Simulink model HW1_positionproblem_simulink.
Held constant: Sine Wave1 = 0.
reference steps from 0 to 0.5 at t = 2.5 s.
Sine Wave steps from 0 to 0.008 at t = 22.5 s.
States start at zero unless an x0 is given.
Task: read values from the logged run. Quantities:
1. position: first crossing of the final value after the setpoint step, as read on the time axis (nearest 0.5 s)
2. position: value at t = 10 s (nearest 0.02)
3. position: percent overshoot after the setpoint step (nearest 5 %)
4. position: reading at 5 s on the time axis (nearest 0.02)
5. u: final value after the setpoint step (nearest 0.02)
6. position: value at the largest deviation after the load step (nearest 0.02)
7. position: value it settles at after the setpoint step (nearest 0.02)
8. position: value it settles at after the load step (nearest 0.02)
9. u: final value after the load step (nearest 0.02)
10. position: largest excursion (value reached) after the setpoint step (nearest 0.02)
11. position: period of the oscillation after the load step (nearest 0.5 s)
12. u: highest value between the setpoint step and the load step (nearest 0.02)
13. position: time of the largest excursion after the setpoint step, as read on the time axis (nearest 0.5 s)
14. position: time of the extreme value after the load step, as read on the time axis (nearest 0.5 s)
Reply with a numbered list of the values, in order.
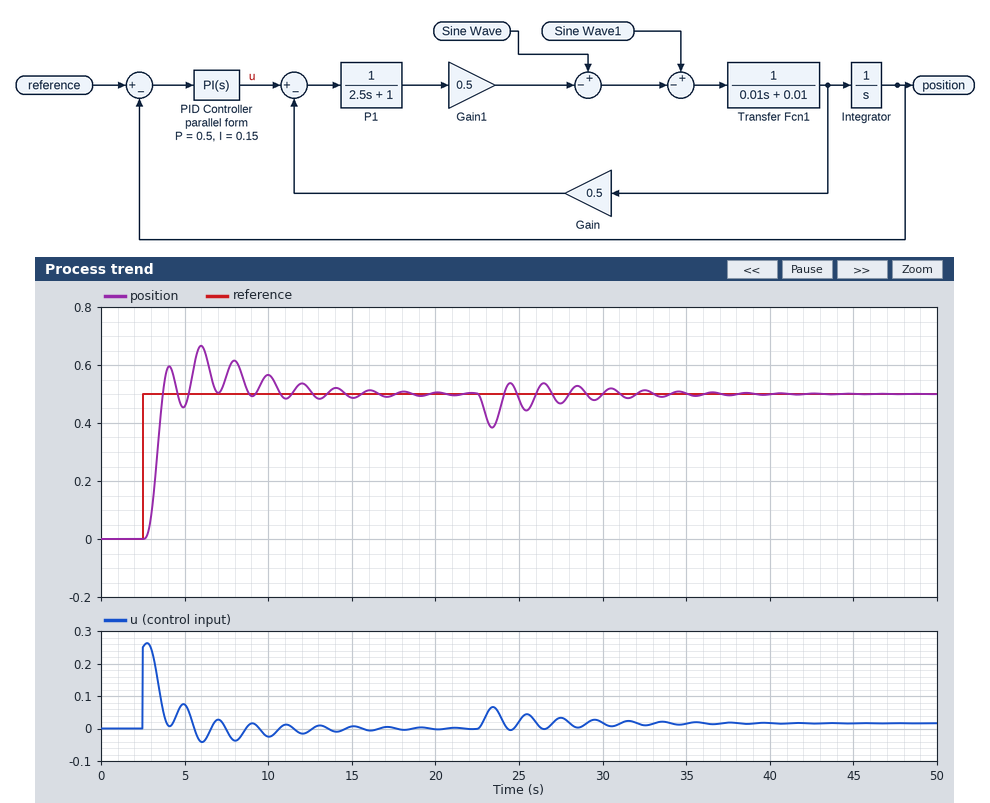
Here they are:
1. 3.5 s
2. 0.56
3. 35 %
4. 0.46
5. 0.00
6. 0.38
7. 0.50
8. 0.50
9. 0.02
10. 0.66
11. 2.0 s
12. 0.26
13. 6.0 s
14. 23.5 s
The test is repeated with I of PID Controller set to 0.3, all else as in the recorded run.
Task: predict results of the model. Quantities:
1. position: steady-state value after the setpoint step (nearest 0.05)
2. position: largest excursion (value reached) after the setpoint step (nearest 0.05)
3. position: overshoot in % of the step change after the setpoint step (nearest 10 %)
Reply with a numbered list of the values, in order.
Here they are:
1. 0.50
2. 0.70
3. 40 %
